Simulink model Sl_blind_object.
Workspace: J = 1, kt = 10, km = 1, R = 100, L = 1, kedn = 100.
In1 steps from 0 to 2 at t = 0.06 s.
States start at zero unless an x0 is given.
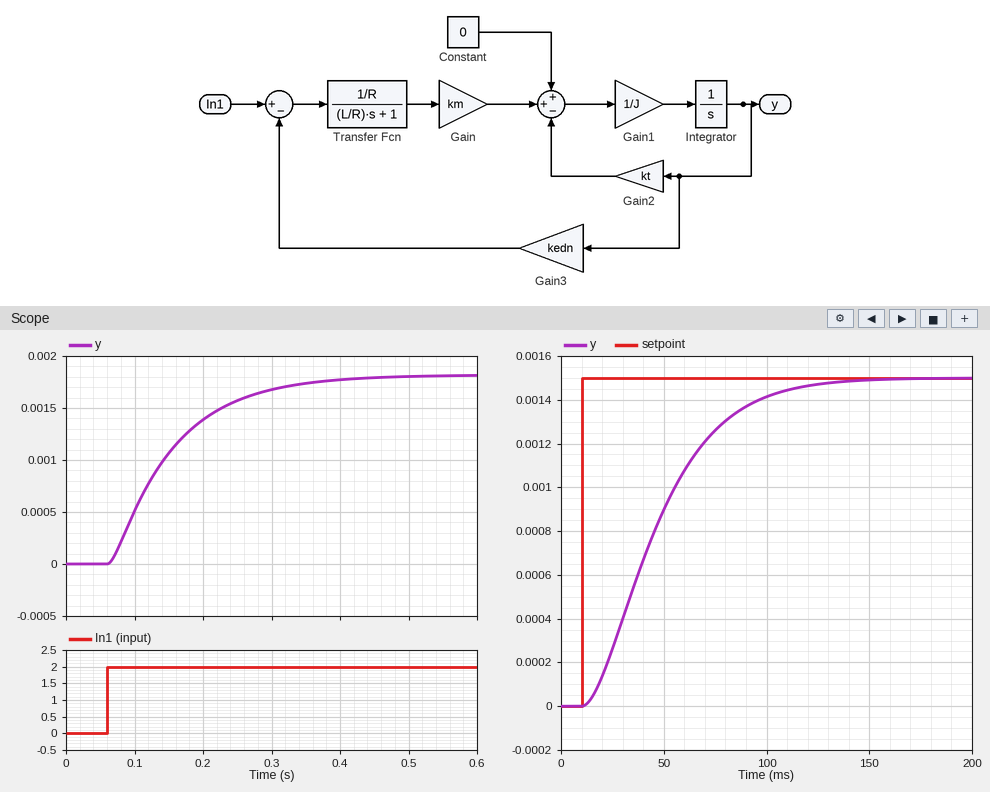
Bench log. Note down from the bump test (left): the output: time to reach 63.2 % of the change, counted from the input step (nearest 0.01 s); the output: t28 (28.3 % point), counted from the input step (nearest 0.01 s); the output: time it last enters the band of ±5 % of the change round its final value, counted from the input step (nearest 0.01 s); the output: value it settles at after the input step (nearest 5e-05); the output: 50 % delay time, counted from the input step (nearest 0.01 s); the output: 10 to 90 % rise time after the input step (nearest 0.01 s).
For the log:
0.10 s
0.04 s
0.28 s
0.00180
0.07 s
0.20 s
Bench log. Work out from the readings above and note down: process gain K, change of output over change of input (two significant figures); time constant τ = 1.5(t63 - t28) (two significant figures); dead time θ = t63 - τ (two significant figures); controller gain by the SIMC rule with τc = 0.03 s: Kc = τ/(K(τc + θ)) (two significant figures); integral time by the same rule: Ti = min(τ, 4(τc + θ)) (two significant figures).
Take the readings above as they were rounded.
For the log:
0.00090
0.090 s
0.010 s
2500
0.090 s
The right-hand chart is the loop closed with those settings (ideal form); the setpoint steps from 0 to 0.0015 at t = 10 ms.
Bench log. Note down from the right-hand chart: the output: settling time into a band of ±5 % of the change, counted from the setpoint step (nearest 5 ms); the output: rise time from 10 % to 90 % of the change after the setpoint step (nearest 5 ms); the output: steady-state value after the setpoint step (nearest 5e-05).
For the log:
95 ms
65 ms
0.00150
